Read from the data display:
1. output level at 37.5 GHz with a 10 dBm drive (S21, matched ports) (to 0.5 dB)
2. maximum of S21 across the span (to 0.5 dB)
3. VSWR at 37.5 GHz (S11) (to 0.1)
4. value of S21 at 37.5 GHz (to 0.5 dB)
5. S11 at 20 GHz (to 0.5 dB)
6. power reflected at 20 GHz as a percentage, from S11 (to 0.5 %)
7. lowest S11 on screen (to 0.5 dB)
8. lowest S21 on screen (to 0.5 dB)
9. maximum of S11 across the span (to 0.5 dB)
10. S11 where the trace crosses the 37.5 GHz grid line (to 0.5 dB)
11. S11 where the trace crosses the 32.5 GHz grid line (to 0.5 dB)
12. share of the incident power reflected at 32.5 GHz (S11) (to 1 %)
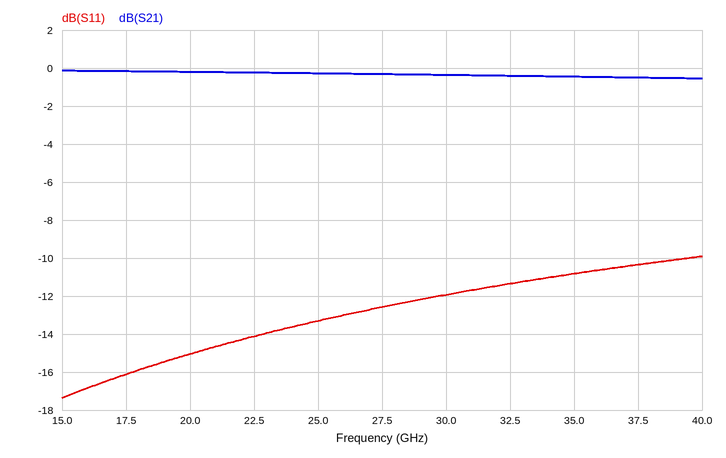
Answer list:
9.5 dBm
0.0 dB
1.9
-0.5 dB
-15.0 dB
3.0 %
-17.5 dB
-0.5 dB
-10.0 dB
-10.5 dB
-11.5 dB
7 %
